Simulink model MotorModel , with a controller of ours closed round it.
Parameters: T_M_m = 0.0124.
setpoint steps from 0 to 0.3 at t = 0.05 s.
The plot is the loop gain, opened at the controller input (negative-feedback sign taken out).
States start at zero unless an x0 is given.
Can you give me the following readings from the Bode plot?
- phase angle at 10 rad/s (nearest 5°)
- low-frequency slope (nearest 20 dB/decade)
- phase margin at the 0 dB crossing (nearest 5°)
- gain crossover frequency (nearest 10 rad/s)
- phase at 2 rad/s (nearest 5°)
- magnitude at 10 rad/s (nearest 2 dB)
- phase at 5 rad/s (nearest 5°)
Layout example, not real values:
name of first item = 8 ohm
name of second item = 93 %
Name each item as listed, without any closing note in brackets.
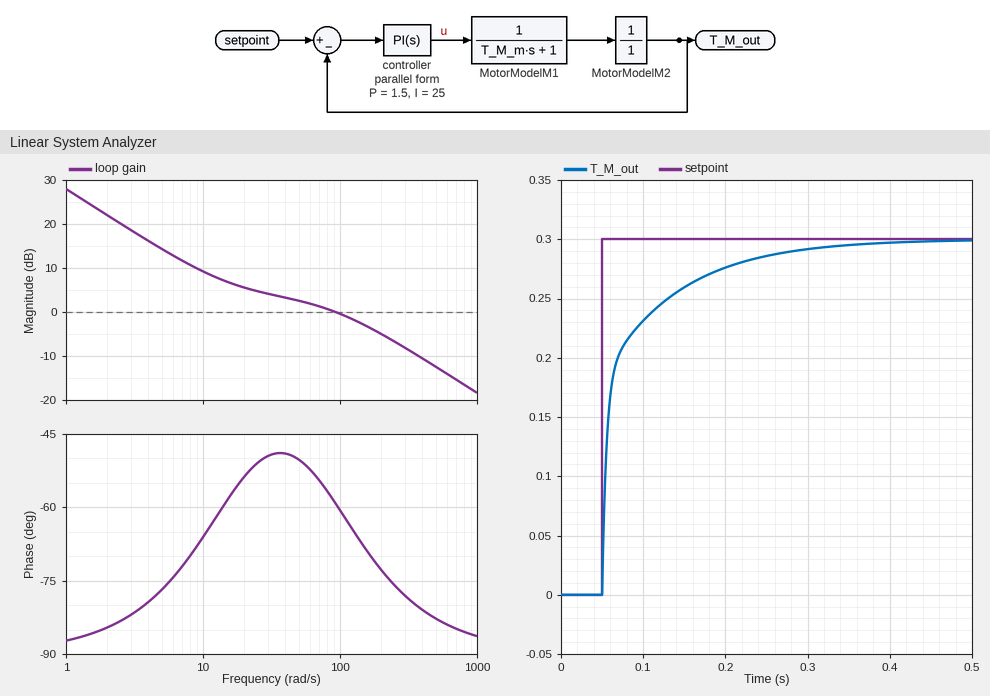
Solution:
phase angle at 10 rad/s = -65°
low-frequency slope = -20 dB/decade
phase margin at the 0 dB crossing = 120°
gain crossover frequency = 90 rad/s
phase at 2 rad/s = -85°
magnitude at 10 rad/s = 10 dB
phase at 5 rad/s = -75°
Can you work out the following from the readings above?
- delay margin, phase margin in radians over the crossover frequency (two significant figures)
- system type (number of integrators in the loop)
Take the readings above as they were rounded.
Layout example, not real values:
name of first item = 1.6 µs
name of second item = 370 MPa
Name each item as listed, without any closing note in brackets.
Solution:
delay margin, phase margin in radians over the crossover frequency = 0.023 s
system type = 1
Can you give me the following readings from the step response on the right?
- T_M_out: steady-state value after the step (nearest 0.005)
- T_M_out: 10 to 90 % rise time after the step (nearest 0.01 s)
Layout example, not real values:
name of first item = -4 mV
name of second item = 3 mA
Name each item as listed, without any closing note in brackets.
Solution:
T_M_out: steady-state value after the step = 0.300
T_M_out: 10 to 90 % rise time after the step = 0.13 s
